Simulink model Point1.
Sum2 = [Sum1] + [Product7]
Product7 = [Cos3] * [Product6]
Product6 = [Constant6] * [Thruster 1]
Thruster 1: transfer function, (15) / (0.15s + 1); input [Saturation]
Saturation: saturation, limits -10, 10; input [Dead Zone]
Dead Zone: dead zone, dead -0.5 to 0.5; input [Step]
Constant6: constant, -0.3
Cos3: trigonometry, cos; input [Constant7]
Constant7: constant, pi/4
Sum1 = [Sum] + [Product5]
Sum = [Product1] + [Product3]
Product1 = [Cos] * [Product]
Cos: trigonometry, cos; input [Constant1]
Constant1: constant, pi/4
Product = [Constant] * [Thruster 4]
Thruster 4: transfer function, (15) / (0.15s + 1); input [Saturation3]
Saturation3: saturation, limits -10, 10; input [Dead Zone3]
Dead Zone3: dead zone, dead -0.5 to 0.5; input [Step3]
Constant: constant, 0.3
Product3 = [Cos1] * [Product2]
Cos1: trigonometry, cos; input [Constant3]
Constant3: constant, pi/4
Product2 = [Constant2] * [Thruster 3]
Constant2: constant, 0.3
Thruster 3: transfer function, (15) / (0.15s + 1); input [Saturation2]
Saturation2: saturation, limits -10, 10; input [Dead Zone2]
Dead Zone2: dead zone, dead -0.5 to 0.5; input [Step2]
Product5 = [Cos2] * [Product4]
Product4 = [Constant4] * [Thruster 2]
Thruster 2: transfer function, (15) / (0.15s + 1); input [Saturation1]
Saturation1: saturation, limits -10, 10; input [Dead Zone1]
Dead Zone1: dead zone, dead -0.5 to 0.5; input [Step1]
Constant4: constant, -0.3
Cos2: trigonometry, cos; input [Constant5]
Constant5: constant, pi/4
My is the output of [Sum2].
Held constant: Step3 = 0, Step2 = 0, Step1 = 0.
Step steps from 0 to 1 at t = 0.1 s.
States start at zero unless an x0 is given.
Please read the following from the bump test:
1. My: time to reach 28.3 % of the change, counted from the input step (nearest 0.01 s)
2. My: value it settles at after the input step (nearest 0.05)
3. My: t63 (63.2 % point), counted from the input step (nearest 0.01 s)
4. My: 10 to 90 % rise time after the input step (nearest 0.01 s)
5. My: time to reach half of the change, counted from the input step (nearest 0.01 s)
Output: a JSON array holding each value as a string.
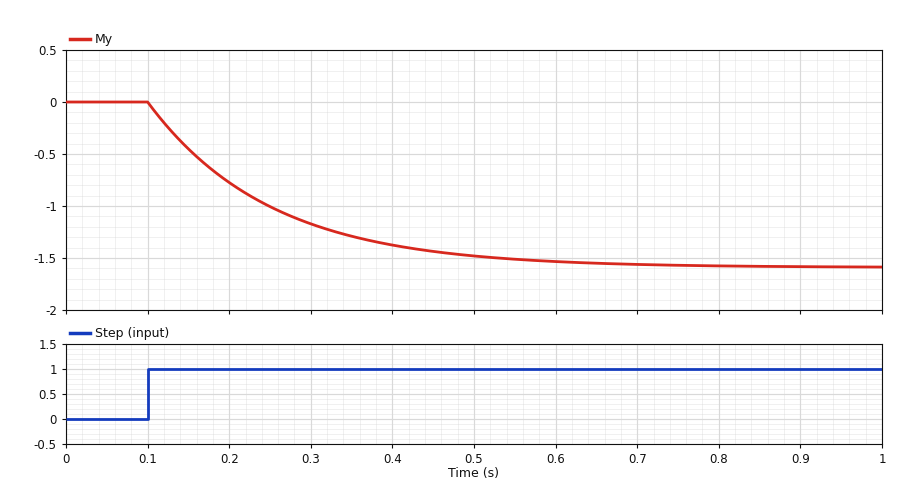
["0.05 s", "-1.60", "0.15 s", "0.33 s", "0.10 s"]
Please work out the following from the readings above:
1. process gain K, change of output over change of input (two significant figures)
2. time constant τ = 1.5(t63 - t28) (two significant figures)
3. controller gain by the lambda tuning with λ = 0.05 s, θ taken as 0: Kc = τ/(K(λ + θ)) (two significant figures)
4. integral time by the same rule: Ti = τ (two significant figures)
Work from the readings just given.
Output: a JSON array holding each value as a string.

["-1.6", "0.15 s", "-1.9", "0.15 s"]
